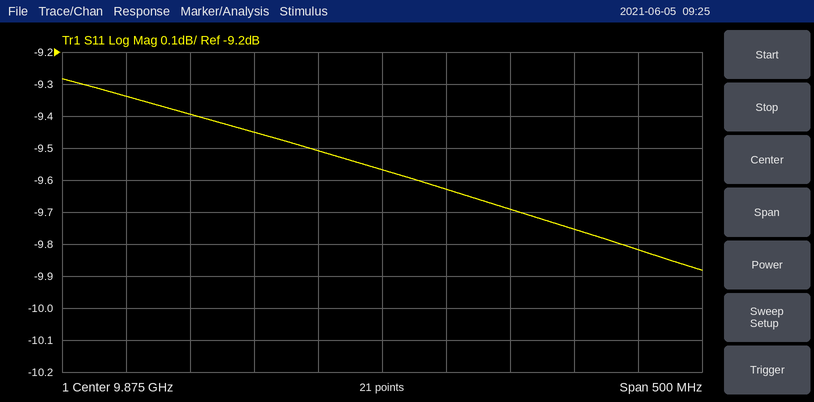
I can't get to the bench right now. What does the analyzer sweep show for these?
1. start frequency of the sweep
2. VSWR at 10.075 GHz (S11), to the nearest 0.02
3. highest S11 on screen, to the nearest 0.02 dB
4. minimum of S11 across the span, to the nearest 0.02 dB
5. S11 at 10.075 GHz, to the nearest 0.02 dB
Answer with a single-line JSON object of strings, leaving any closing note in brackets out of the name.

{"start frequency of the sweep": "9.625 GHz", "VSWR at 10.075 GHz (S11), to the nearest 0.02": "1.96", "highest S11 on screen, to the nearest 0.02 dB": "-9.28 dB", "minimum of S11 across the span, to the nearest 0.02 dB": "-9.88 dB", "S11 at 10.075 GHz, to the nearest 0.02 dB": "-9.82 dB"}
